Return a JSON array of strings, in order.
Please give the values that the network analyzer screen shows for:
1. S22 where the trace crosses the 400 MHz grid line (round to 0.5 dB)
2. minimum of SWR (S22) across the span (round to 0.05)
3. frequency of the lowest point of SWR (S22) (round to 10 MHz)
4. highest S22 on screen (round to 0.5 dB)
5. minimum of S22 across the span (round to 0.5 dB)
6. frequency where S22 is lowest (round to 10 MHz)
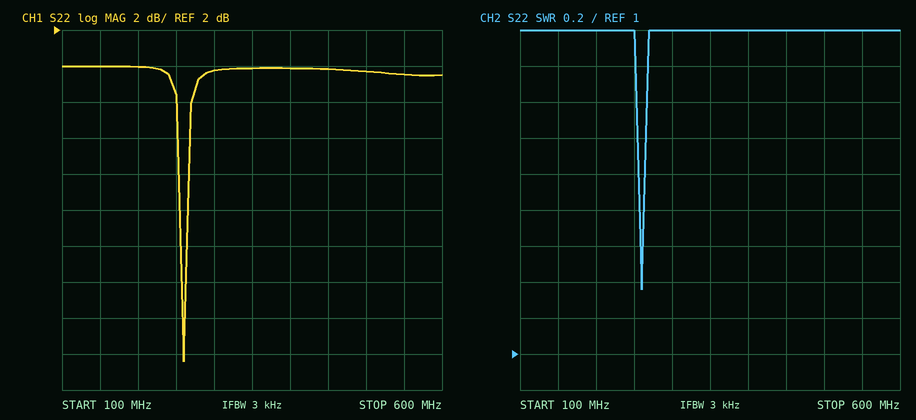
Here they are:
["0.0 dB", "1.35", "260 MHz", "0.0 dB", "-16.5 dB", "260 MHz"]
